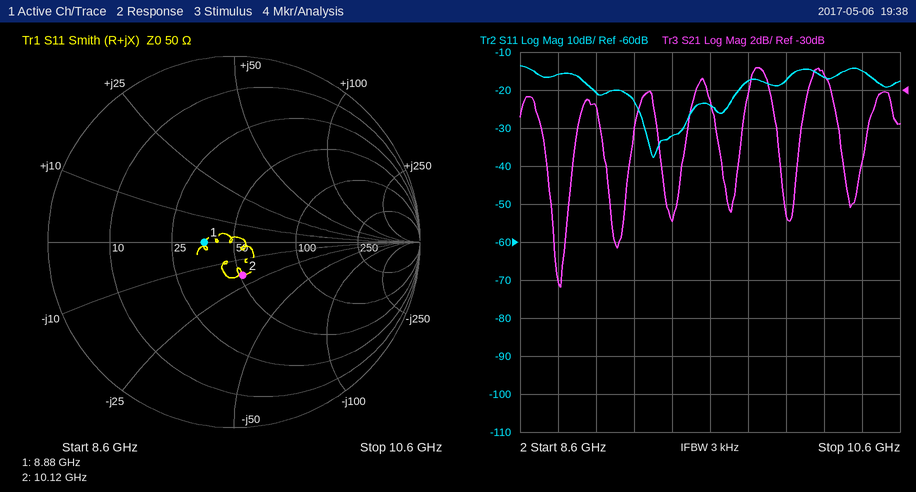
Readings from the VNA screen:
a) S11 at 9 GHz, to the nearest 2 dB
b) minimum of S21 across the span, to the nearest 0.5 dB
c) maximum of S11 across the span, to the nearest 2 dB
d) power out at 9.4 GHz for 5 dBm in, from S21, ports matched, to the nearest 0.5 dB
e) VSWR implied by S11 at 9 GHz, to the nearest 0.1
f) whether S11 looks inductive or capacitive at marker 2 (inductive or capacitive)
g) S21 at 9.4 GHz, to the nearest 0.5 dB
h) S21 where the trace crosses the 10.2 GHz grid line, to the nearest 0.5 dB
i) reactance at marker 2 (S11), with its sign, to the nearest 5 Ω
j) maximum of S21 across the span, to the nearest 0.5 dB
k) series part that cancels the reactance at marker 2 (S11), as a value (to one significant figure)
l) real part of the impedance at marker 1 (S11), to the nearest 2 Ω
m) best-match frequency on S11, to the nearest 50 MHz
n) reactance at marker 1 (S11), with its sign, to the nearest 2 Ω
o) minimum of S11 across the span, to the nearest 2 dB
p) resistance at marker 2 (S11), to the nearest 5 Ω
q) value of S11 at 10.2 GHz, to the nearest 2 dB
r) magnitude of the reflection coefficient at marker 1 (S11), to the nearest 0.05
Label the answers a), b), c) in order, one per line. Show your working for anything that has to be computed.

a) -20 dB
b) -40.5 dB
c) -14 dB
d) 5 dBm + (-37.0 dB) = -32.0 dBm
e) |Γ| = 10^(-20/20) = 0.1000; VSWR = (1 + 0.1000)/(1 − 0.1000) ≈ 1.2
f) capacitive
g) -37.0 dB
h) -29.0 dB
i) -20 Ω
j) -29.0 dB
k) L = 20 Ω/(2π × 10.12 GHz) ≈ 315 pH, so 300 pH to one significant figure
l) 36 Ω
m) 9.30 GHz
n) 0 Ω
o) -38 dB
p) 50 Ω
q) -16 dB
r) 0.15
